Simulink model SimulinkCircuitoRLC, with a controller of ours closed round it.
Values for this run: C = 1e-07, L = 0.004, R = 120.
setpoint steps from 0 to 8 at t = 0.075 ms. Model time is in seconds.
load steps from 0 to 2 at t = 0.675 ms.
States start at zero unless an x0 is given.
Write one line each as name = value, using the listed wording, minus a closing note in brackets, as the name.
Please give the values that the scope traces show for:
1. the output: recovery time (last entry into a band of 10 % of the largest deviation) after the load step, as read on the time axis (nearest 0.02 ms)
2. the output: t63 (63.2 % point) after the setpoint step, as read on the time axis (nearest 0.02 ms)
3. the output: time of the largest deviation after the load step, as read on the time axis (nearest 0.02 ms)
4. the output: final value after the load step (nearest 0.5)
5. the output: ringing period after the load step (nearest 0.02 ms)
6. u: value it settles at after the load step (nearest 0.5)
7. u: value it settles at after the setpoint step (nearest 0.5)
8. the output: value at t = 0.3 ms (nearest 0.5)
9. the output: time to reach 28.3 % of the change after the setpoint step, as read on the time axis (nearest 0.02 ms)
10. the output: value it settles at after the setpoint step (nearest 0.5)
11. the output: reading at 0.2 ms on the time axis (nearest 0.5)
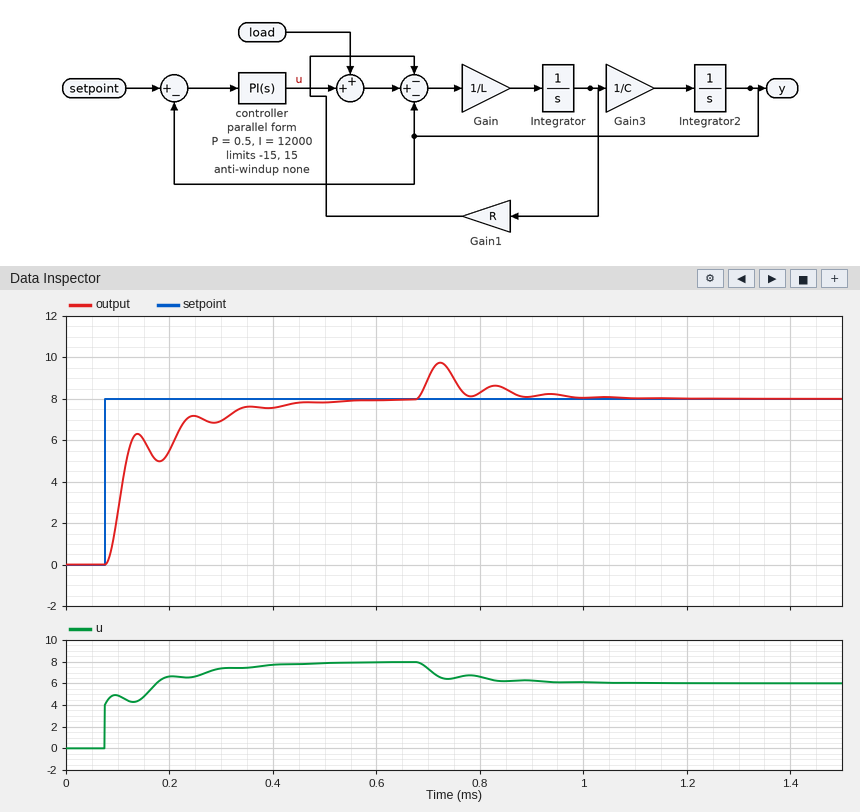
the output: recovery time (last entry into a band of 10 % of the largest deviation) after the load step, as read on the time axis = 0.96 ms
the output: t63 (63.2 % point) after the setpoint step, as read on the time axis = 0.12 ms
the output: time of the largest deviation after the load step, as read on the time axis = 0.72 ms
the output: final value after the load step = 8.0
the output: ringing period after the load step = 0.10 ms
u: value it settles at after the load step = 6.0
u: value it settles at after the setpoint step = 8.0
the output: value at t = 0.3 ms = 7.0
the output: time to reach 28.3 % of the change after the setpoint step, as read on the time axis = 0.10 ms
the output: value it settles at after the setpoint step = 8.0
the output: reading at 0.2 ms on the time axis = 5.5
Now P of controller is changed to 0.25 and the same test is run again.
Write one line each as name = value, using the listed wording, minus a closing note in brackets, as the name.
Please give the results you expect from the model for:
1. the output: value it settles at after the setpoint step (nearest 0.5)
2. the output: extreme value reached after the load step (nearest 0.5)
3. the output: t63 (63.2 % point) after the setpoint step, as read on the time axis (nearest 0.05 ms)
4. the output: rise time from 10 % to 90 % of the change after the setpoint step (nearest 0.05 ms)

the output: value it settles at after the setpoint step = 8.0
the output: extreme value reached after the load step = 10.0
the output: t63 (63.2 % point) after the setpoint step, as read on the time axis = 0.15 ms
the output: rise time from 10 % to 90 % of the change after the setpoint step = 0.15 ms
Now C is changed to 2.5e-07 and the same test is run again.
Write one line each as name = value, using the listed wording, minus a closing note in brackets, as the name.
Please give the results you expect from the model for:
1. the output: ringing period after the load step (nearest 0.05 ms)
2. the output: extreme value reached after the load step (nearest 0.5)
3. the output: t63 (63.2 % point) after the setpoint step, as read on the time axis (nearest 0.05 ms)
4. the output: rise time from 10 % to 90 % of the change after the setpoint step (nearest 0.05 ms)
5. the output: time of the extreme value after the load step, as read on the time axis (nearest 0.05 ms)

the output: ringing period after the load step = 0.20 ms
the output: extreme value reached after the load step = 9.5
the output: t63 (63.2 % point) after the setpoint step, as read on the time axis = 0.15 ms
the output: rise time from 10 % to 90 % of the change after the setpoint step = 0.20 ms
the output: time of the extreme value after the load step, as read on the time axis = 0.75 ms
